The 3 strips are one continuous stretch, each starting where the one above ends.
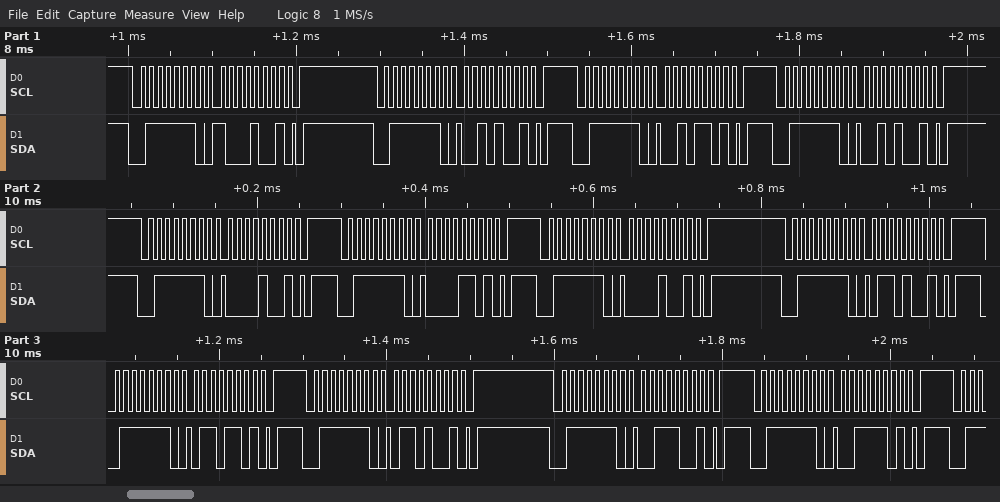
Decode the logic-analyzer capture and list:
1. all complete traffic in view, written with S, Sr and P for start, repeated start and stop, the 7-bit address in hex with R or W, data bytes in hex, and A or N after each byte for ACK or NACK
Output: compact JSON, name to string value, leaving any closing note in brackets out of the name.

{"all complete traffic in view, written with S, Sr and P for start, repeated start and stop, the 7-bit address in hex with R or W, data bytes in hex, and A or N after each byte for ACK or NACK": "S 3FW A 89 A P S 3FW A 29 A P S 3FW A 2D A P S 3FW A 29 A P S 3FW A 09 A P S 3FW A 0D A P S 3FW A 09 A P S 3FW A 69 A P S 3FW A 6D A P S 3FW A 69 A P S 3FW A 39 A P S 3FW A 3D A P"}
